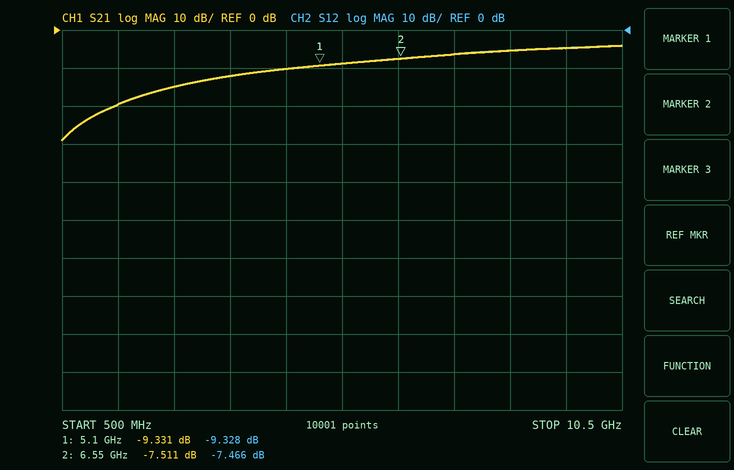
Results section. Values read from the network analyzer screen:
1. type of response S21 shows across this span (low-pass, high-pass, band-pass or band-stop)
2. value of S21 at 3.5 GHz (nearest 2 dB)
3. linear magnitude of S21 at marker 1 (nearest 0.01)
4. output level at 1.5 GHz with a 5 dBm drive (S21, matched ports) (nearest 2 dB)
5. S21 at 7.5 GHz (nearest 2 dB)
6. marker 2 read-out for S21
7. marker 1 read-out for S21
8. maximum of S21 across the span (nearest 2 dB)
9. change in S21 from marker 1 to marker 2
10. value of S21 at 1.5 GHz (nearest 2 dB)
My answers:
high-pass
-12 dB
0.34
-14 dBm
-6 dB
-7.511 dB
-9.331 dB
-4 dB
1.820 dB
-20 dB
